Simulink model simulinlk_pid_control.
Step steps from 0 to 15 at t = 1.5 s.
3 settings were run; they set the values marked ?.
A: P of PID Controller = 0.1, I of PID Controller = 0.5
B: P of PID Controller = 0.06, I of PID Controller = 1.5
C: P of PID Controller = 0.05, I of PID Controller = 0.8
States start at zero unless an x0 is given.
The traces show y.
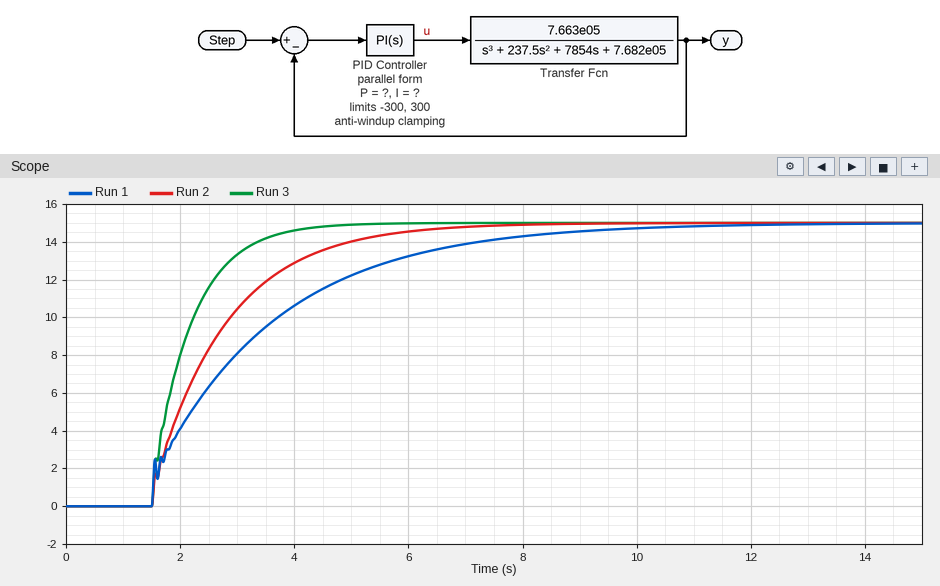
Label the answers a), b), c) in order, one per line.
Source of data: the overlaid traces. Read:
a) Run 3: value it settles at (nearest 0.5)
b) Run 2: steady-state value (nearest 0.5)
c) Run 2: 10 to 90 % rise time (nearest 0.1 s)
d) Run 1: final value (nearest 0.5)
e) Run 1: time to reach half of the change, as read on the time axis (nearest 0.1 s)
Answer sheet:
a) 15.0
b) 15.0
c) 2.9 s
d) 15.0
e) 2.8 s
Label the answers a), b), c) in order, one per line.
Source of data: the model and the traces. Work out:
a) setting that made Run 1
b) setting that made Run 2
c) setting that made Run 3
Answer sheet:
a) A
b) C
c) B
